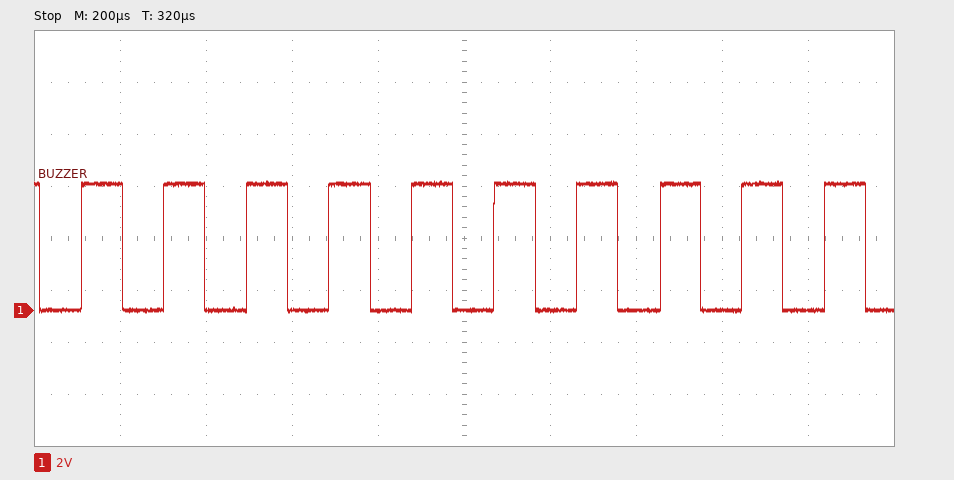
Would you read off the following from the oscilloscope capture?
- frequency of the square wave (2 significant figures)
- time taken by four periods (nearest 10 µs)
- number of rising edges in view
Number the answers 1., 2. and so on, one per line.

1. 5.2 kHz
2. 770 µs
3. 10
